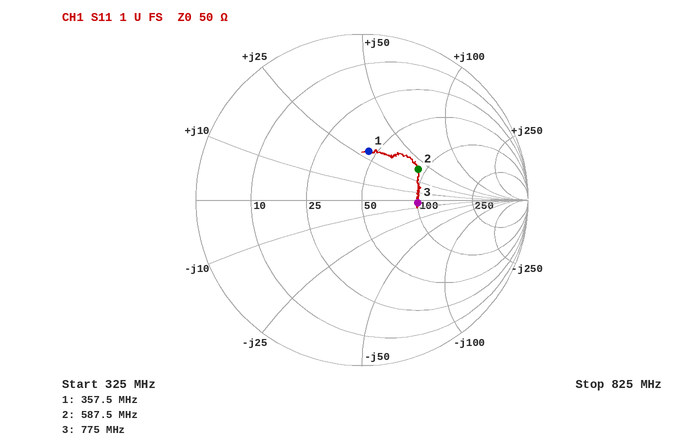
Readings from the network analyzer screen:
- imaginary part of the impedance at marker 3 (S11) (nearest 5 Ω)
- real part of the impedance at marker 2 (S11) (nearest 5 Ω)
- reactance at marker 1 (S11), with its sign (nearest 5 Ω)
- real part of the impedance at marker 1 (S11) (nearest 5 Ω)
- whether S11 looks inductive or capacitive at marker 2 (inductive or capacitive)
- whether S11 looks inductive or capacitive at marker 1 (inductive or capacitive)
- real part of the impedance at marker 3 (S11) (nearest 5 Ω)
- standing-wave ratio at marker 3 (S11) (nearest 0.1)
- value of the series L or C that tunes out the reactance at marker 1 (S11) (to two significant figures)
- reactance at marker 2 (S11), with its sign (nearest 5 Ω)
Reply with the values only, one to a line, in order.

-5 Ω
90 Ω
+30 Ω
45 Ω
inductive
inductive
100 Ω
2.0
15 pF
+40 Ω
